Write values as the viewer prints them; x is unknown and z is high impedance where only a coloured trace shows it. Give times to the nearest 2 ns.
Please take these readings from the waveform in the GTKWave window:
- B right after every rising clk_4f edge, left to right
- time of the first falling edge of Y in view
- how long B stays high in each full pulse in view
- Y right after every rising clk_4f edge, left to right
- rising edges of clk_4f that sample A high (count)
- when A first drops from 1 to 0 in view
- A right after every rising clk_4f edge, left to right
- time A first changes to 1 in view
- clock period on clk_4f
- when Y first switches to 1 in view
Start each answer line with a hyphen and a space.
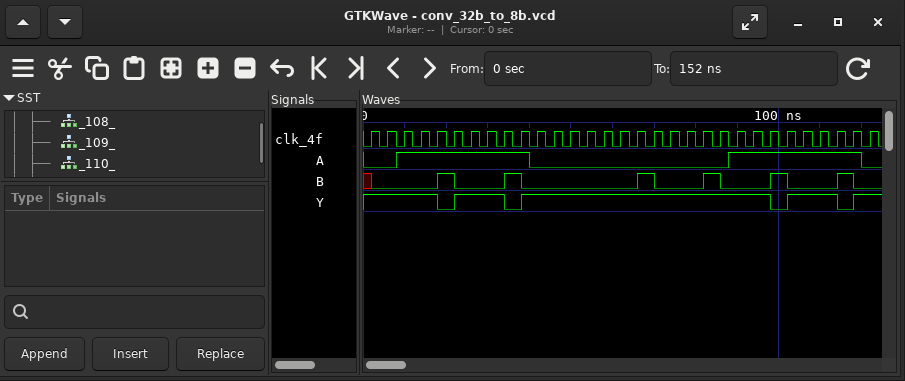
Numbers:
- 0 0 0 0 1 0 0 0 1 0 0 0 0 0 0 0 1 0 0 0 1 0 0 0 1 0 0 0 1 0 0
- 18 ns
- 4 ns, 4 ns, 4 ns, 4 ns, 4 ns, 4 ns
- 1 1 1 1 0 1 1 1 0 1 1 1 1 1 1 1 1 1 1 1 1 1 1 1 0 1 1 1 0 1 1
- 16
- 40 ns
- 0 0 1 1 1 1 1 1 1 1 0 0 0 0 0 0 0 0 0 0 0 0 1 1 1 1 1 1 1 1 0
- 8 ns
- 4 ns
- 22 ns
